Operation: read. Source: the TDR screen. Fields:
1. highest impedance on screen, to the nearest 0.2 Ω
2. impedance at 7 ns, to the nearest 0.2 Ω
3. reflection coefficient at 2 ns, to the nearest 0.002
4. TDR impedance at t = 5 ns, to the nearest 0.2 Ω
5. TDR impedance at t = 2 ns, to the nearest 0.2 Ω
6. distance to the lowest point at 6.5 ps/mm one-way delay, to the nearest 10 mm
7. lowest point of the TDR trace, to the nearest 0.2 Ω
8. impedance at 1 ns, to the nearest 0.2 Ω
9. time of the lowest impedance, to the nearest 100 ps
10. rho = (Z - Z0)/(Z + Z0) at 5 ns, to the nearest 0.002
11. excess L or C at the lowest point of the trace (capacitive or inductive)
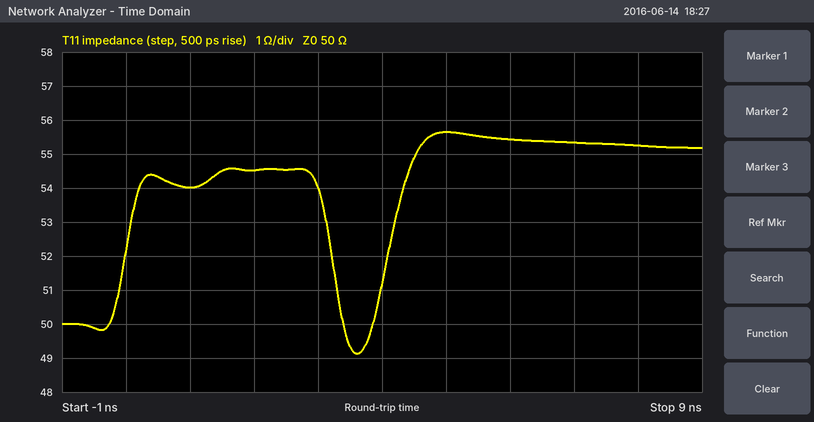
55.6 Ω
55.4 Ω
+0.044
55.6 Ω
54.6 Ω
280 mm
49.2 Ω
54.0 Ω
3.6 ns
+0.054
capacitive
